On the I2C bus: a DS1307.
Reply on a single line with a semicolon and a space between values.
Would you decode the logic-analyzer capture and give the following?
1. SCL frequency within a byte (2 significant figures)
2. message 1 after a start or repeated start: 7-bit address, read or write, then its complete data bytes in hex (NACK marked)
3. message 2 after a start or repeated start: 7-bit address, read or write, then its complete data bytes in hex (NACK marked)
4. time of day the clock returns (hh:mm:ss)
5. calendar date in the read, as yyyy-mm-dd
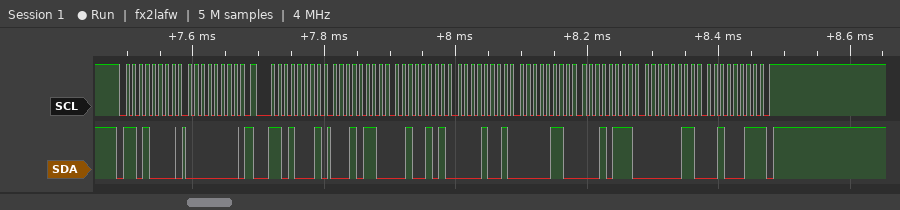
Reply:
100 kHz; 0x68 write: 00; 0x68 read: 16 25 09 06 17 03 23 NACK; 09:25:16; 2023-03-17
